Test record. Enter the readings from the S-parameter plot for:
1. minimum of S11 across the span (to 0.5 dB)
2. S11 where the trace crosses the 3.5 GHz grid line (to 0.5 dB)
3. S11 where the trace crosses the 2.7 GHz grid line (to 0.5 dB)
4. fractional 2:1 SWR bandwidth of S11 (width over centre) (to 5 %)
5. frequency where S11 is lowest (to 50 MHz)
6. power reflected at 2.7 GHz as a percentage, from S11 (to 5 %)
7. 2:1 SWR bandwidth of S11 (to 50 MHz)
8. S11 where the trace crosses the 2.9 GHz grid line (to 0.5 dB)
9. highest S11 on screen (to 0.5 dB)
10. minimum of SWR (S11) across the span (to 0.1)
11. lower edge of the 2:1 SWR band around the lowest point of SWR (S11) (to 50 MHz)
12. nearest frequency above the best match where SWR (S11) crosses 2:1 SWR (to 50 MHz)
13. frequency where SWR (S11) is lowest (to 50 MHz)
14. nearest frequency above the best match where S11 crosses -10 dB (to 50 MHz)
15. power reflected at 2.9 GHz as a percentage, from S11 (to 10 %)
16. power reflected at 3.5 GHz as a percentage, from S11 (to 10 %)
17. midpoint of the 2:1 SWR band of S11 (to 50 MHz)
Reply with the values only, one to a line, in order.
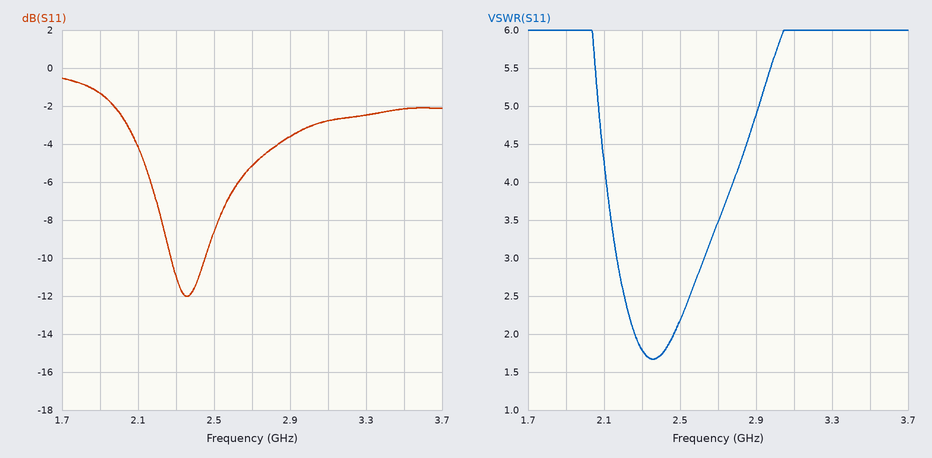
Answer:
-12.0 dB
-2.0 dB
-5.0 dB
10 %
2.35 GHz
30 %
200 MHz
-3.5 dB
-0.5 dB
1.7
2.25 GHz
2.45 GHz
2.35 GHz
2.45 GHz
40 %
60 %
2.35 GHz
